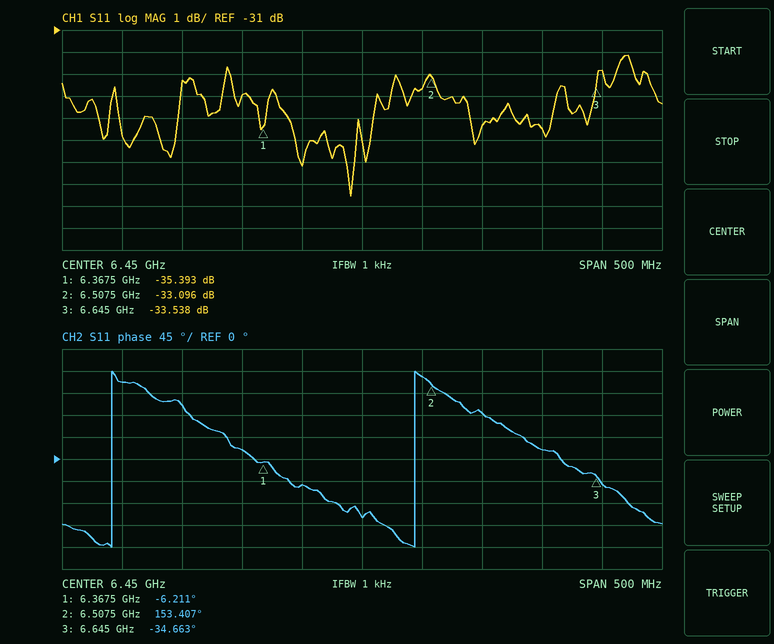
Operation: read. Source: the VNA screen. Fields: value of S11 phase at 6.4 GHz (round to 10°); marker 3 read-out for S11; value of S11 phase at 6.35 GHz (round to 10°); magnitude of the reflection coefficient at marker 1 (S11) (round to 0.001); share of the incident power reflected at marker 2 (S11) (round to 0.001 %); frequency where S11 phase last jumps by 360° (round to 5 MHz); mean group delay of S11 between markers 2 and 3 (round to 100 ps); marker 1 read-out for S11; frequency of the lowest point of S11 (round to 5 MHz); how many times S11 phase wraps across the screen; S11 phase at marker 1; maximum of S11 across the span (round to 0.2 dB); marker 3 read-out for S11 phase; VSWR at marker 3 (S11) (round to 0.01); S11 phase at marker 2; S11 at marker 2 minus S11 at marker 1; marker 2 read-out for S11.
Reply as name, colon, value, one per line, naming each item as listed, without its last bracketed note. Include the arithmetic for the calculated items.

value of S11 phase at 6.4 GHz: -50°
marker 3 read-out for S11: -33.538 dB
value of S11 phase at 6.35 GHz: 20°
magnitude of the reflection coefficient at marker 1 (S11): 10^(-35.393/20) ≈ 0.017
share of the incident power reflected at marker 2 (S11): 10^(-33.096/10) ≈ 0.049 %
frequency where S11 phase last jumps by 360°: 6.495 GHz
mean group delay of S11 between markers 2 and 3: −(-34.663° − (153.407°))/(360° × 137.5 MHz) ≈ 3.8 ns
marker 1 read-out for S11: -35.393 dB
frequency of the lowest point of S11: 6.440 GHz
how many times S11 phase wraps across the screen: 2
S11 phase at marker 1: -6.211°
maximum of S11 across the span: -32.2 dB
marker 3 read-out for S11 phase: -34.663°
VSWR at marker 3 (S11): (1 + 0.0210)/(1 − 0.0210) ≈ 1.04
S11 phase at marker 2: 153.407°
S11 at marker 2 minus S11 at marker 1: -33.096 − (-35.393) = 2.297 dB
marker 2 read-out for S11: -33.096 dB
